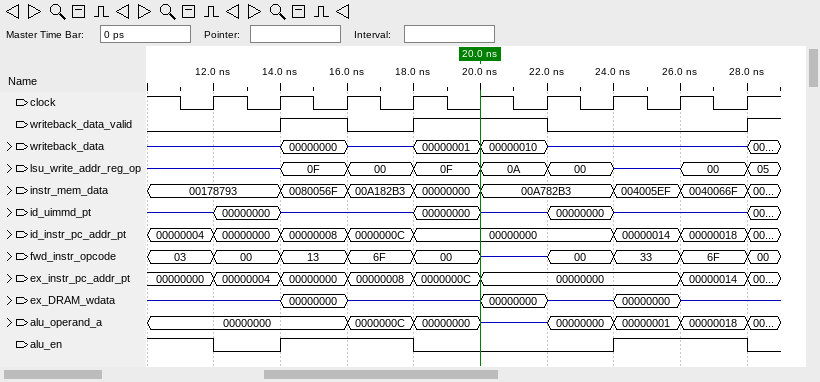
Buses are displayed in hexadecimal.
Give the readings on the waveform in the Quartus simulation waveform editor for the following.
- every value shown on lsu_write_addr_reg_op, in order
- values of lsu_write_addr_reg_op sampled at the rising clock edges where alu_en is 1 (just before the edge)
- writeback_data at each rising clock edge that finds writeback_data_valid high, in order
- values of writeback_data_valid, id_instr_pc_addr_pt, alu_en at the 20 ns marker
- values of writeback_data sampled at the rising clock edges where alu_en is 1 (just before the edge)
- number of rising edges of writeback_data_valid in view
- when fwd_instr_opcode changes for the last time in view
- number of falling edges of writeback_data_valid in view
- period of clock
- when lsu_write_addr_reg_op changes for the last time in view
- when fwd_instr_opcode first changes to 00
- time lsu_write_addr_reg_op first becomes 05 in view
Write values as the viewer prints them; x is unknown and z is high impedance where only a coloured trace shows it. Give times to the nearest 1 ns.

z, 0F, 00, 0F, 0A, 00, z, 00, 05
z, 0F, 00, z, 00
00000000, 00000001, 00000010
writeback_data_valid=1, id_instr_pc_addr_pt=00000000, alu_en=0
z, 00000000, z, z, z
3
28 ns
2
2 ns
28 ns
12 ns
28 ns
